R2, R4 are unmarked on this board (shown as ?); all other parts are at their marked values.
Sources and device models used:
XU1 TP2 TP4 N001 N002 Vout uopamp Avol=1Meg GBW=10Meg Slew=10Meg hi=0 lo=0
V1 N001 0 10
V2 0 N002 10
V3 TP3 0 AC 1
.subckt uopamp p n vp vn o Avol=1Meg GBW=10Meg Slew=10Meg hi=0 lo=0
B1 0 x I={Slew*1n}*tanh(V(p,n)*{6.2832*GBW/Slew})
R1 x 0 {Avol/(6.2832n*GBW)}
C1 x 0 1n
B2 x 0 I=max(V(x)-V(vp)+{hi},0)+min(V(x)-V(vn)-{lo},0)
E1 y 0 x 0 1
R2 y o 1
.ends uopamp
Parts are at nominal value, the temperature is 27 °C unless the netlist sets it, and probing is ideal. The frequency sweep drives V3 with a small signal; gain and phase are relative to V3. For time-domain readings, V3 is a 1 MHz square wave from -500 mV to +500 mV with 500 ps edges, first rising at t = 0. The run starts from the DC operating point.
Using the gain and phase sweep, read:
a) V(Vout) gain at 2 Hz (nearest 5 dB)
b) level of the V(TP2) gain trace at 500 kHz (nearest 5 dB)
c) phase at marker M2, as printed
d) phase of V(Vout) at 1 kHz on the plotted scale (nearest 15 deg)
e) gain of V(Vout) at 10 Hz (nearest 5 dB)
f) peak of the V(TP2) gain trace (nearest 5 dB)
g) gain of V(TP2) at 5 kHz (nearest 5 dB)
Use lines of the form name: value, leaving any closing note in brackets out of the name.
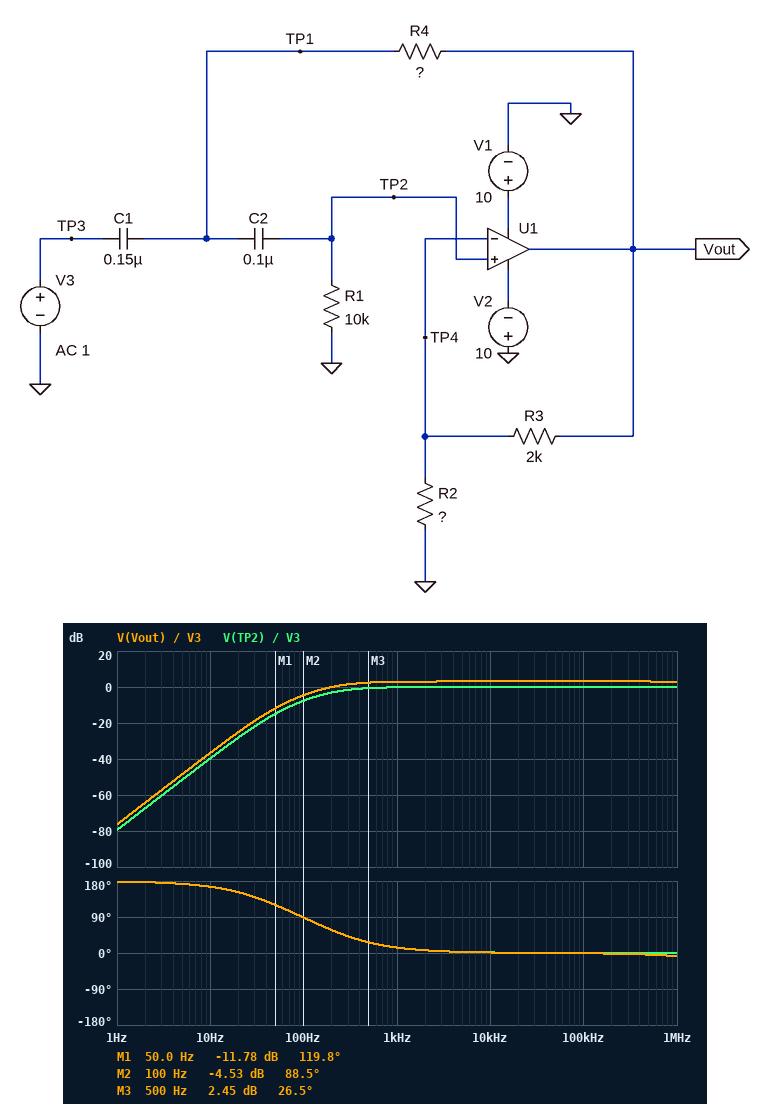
V(Vout) gain at 2 Hz: -65 dB
level of the V(TP2) gain trace at 500 kHz: 0 dB
phase at marker M2, as printed: 88.5 deg
phase of V(Vout) at 1 kHz on the plotted scale: 15 deg
gain of V(Vout) at 10 Hz: -35 dB
peak of the V(TP2) gain trace: 0 dB
gain of V(TP2) at 5 kHz: 0 dB
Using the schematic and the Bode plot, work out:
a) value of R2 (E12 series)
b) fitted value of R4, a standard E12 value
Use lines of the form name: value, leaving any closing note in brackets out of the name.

value of R2: 4.7 kΩ
fitted value of R4, a standard E12 value: 18 kΩ
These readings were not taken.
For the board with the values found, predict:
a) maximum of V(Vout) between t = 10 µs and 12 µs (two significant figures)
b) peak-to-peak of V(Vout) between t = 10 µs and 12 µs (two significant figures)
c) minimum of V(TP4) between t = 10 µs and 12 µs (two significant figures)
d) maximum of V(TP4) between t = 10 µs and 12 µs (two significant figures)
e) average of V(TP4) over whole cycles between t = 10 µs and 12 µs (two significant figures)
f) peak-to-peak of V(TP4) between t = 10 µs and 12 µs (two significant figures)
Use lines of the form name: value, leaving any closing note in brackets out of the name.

maximum of V(Vout) between t = 10 µs and 12 µs: 1.4 V
peak-to-peak of V(Vout) between t = 10 µs and 12 µs: 1.4 V
minimum of V(TP4) between t = 10 µs and 12 µs: -9.0 mV
maximum of V(TP4) between t = 10 µs and 12 µs: 990 mV
average of V(TP4) over whole cycles between t = 10 µs and 12 µs: 490 mV
peak-to-peak of V(TP4) between t = 10 µs and 12 µs: 1.0 V
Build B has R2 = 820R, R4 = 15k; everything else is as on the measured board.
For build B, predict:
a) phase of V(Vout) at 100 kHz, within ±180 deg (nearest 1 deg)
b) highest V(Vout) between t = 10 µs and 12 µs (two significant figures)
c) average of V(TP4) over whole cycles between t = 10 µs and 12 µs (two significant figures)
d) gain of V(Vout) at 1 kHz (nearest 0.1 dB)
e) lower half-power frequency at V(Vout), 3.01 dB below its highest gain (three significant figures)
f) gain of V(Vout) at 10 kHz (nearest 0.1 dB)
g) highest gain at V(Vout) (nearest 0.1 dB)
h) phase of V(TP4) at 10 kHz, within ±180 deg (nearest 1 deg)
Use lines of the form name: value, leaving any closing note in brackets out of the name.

phase of V(Vout) at 100 kHz, within ±180 deg: -2 deg
highest V(Vout) between t = 10 µs and 12 µs: 3.4 V
average of V(TP4) over whole cycles between t = 10 µs and 12 µs: 500 mV
gain of V(Vout) at 1 kHz: 10.8 dB
lower half-power frequency at V(Vout), 3.01 dB below its highest gain: 89.5 Hz
gain of V(Vout) at 10 kHz: 10.7 dB
highest gain at V(Vout): 12.8 dB
phase of V(TP4) at 10 kHz, within ±180 deg: 0 deg
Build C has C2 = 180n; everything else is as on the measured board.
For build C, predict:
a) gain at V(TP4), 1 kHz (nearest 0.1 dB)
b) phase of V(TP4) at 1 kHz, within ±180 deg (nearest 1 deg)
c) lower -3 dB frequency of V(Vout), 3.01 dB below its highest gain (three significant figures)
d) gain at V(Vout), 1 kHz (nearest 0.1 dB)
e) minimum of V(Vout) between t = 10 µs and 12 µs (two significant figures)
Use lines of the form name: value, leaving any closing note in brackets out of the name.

gain at V(TP4), 1 kHz: -0.1 dB
phase of V(TP4) at 1 kHz, within ±180 deg: 10 deg
lower -3 dB frequency of V(Vout), 3.01 dB below its highest gain: 140 Hz
gain at V(Vout), 1 kHz: 3.0 dB
minimum of V(Vout) between t = 10 µs and 12 µs: -9.1 mV
